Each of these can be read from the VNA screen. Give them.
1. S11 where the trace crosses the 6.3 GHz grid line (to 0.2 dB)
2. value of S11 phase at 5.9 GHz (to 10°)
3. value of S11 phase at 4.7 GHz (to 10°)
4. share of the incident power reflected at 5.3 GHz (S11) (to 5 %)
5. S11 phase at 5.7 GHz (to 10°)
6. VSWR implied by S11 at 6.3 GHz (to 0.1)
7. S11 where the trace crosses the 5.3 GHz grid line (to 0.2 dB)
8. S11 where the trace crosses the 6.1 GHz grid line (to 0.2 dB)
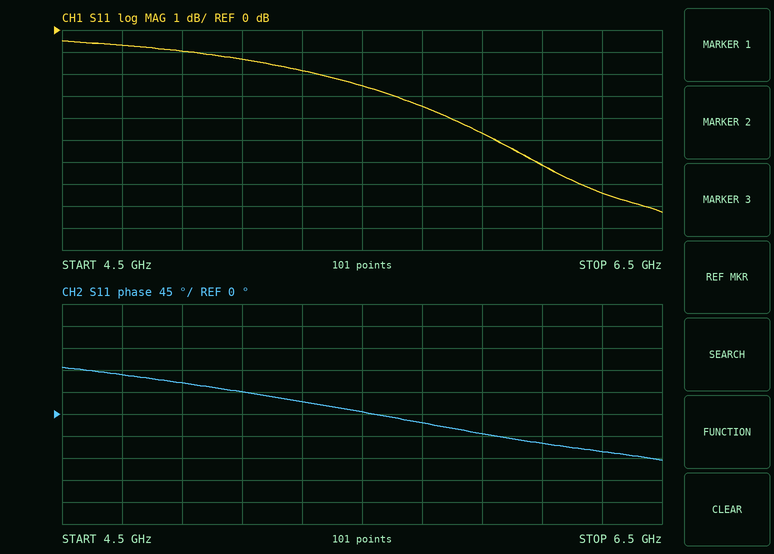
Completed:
-7.4 dB
-40°
80°
65 %
-20°
2.5
-1.8 dB
-6.2 dB
